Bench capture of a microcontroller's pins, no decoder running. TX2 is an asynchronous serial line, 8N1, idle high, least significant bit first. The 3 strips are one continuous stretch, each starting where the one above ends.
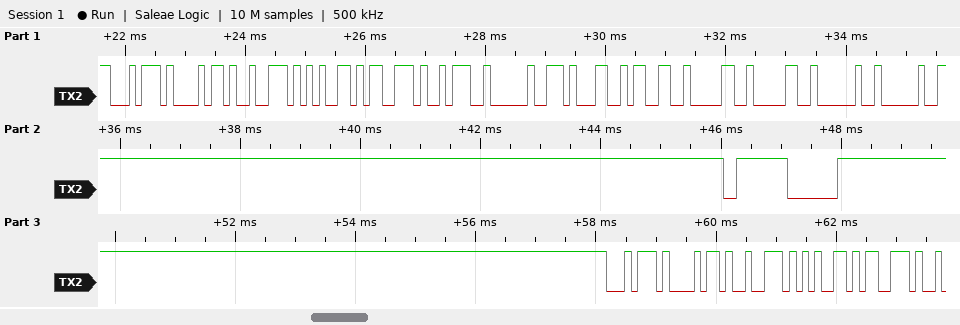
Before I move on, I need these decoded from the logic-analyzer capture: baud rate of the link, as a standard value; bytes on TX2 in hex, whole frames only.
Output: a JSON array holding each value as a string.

["9600 baud", "74 68 72 65 73 3A 20 31 33 30 30 20 20 FE 80 74 68 72 65 73"]
